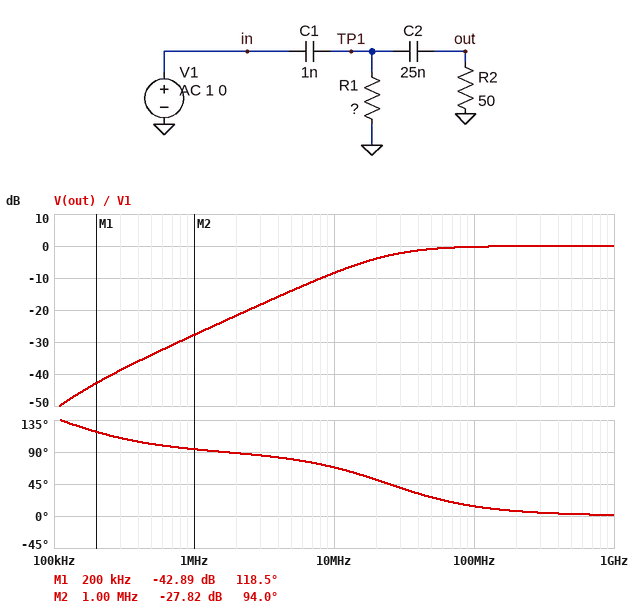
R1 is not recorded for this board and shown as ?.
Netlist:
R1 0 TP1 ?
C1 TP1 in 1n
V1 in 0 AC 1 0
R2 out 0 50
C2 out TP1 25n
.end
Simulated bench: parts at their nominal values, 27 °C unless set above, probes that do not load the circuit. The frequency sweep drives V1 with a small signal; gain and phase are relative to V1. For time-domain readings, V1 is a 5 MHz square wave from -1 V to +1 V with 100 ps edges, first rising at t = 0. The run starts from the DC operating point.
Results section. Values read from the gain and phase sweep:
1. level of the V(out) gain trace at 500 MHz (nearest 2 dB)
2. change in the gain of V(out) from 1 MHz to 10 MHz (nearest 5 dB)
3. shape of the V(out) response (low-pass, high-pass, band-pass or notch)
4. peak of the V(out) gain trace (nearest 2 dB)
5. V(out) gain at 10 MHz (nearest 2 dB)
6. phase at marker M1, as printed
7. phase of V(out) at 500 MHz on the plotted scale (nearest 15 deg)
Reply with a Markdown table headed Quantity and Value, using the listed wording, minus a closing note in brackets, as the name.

| Quantity | Value |
|---|---|
| level of the V(out) gain trace at 500 MHz | 0 dB |
| change in the gain of V(out) from 1 MHz to 10 MHz | 20 dB |
| shape of the V(out) response | high-pass |
| peak of the V(out) gain trace | 0 dB |
| V(out) gain at 10 MHz | -8 dB |
| phase at marker M1, as printed | 118.5 deg |
| phase of V(out) at 500 MHz on the plotted scale | 0 deg |
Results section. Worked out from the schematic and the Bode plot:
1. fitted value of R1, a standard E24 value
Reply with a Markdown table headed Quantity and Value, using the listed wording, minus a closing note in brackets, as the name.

| Quantity | Value |
|---|---|
| fitted value of R1, a standard E24 value | 7.5 Ω |
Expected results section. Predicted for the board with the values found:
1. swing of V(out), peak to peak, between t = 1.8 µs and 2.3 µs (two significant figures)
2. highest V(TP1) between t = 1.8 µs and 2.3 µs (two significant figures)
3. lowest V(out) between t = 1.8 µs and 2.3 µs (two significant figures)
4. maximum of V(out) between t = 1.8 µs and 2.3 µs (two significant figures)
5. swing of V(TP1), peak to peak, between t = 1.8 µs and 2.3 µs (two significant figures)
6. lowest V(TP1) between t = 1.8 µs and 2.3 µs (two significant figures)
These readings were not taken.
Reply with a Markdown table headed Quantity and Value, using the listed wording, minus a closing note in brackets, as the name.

| Quantity | Value |
|---|---|
| swing of V(out), peak to peak, between t = 1.8 µs and 2.3 µs | 4.0 V |
| highest V(TP1) between t = 1.8 µs and 2.3 µs | 2.0 V |
| lowest V(out) between t = 1.8 µs and 2.3 µs | -2.0 V |
| maximum of V(out) between t = 1.8 µs and 2.3 µs | 2.0 V |
| swing of V(TP1), peak to peak, between t = 1.8 µs and 2.3 µs | 4.0 V |
| lowest V(TP1) between t = 1.8 µs and 2.3 µs | -2.0 V |
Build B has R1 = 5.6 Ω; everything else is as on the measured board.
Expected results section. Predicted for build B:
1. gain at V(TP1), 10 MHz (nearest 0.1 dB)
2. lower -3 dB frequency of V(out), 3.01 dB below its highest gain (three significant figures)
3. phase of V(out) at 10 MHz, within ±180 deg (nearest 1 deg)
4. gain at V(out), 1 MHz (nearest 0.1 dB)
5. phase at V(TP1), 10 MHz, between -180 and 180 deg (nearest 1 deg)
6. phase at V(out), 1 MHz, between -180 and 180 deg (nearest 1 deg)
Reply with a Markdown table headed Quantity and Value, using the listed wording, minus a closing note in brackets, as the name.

| Quantity | Value |
|---|---|
| gain at V(TP1), 10 MHz | -10.4 dB |
| lower -3 dB frequency of V(out), 3.01 dB below its highest gain | 31.6 MHz |
| phase of V(out) at 10 MHz, within ±180 deg | 73 deg |
| gain at V(out), 1 MHz | -30.1 dB |
| phase at V(TP1), 10 MHz, between -180 and 180 deg | 72 deg |
| phase at V(out), 1 MHz, between -180 and 180 deg | 95 deg |
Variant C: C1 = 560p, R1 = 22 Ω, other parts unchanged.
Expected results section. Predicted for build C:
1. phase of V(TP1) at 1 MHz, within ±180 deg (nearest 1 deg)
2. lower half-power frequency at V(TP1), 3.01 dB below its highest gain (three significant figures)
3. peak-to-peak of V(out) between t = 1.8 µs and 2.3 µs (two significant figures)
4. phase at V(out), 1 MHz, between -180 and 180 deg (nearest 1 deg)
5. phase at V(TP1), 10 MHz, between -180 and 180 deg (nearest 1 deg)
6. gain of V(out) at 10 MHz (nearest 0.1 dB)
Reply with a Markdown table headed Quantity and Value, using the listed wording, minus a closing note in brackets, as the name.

| Quantity | Value |
|---|---|
| phase of V(TP1) at 1 MHz, within ±180 deg | 85 deg |
| lower half-power frequency at V(TP1), 3.01 dB below its highest gain | 18.6 MHz |
| peak-to-peak of V(out) between t = 1.8 µs and 2.3 µs | 4.0 V |
| phase at V(out), 1 MHz, between -180 and 180 deg | 92 deg |
| phase at V(TP1), 10 MHz, between -180 and 180 deg | 62 deg |
| gain of V(out) at 10 MHz | -6.5 dB |
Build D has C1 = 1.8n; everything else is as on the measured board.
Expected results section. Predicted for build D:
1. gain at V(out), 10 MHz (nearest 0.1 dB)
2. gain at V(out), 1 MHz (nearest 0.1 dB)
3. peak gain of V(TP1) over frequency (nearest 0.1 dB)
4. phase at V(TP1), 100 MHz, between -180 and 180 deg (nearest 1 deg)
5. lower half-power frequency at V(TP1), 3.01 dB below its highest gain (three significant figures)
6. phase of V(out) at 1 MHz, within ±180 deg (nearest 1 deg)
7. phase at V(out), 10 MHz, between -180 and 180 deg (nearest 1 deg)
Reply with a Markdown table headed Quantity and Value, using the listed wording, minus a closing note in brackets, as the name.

| Quantity | Value |
|---|---|
| gain at V(out), 10 MHz | -4.5 dB |
| gain at V(out), 1 MHz | -22.7 dB |
| peak gain of V(TP1) over frequency | 0 dB |
| phase at V(TP1), 100 MHz, between -180 and 180 deg | 8 deg |
| lower half-power frequency at V(TP1), 3.01 dB below its highest gain | 13.6 MHz |
| phase of V(out) at 1 MHz, within ±180 deg | 92 deg |
| phase at V(out), 10 MHz, between -180 and 180 deg | 54 deg |
